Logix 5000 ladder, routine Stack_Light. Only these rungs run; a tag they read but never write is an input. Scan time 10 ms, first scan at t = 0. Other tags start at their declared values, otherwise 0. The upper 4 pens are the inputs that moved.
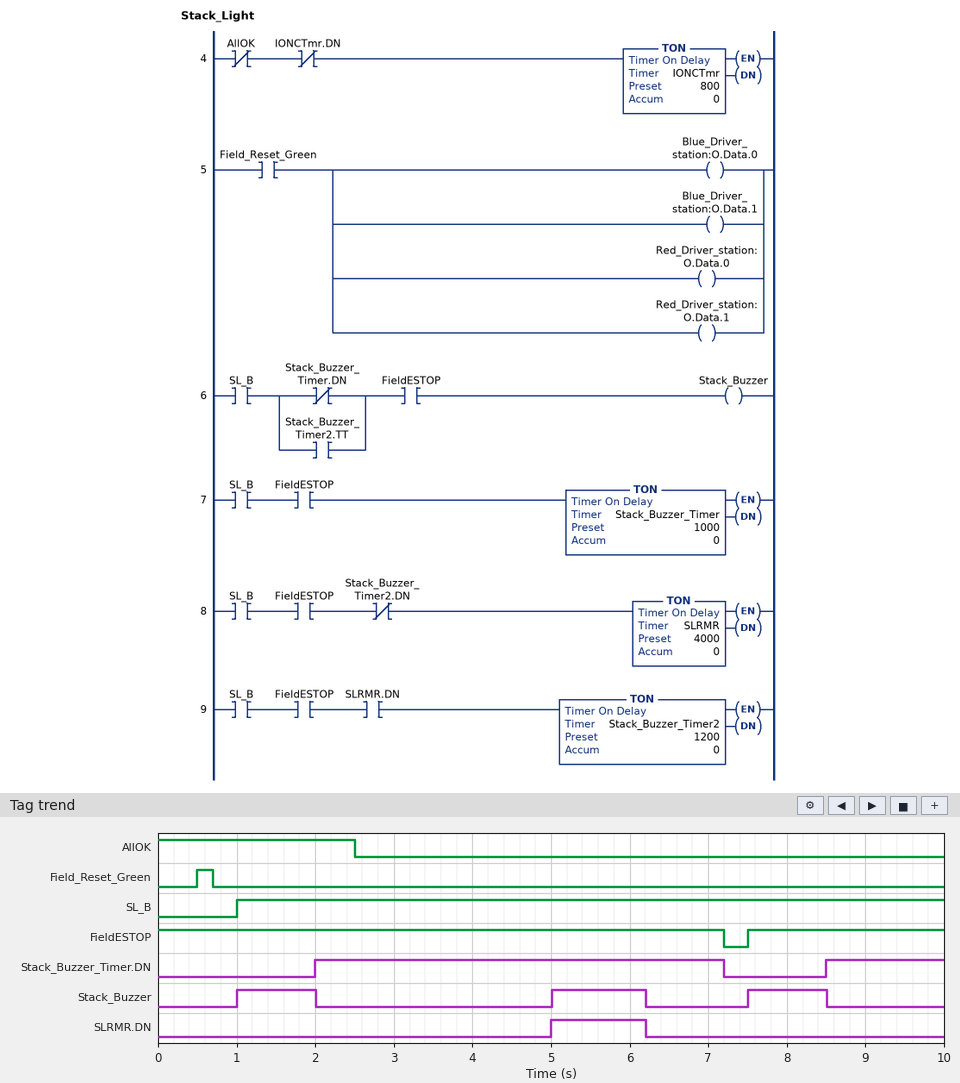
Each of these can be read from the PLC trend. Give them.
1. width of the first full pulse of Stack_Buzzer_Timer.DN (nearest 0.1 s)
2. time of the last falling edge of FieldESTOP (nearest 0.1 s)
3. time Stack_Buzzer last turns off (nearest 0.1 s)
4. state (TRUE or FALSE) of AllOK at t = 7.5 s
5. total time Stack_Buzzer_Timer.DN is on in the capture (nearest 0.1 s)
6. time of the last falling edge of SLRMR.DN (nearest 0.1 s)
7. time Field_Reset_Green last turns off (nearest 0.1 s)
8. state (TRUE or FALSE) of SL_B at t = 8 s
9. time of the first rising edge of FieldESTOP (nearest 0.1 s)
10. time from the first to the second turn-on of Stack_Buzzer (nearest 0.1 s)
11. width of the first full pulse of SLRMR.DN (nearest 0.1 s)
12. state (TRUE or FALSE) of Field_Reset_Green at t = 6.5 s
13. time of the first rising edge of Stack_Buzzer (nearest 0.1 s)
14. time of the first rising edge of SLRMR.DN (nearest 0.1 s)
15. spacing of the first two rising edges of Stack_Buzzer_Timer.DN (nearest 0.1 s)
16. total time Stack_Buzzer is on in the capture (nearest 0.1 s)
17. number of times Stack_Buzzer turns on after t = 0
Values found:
5.2 s
7.2 s
8.5 s
FALSE
6.7 s
6.2 s
0.7 s
TRUE
7.5 s
4.0 s
1.2 s
FALSE
1.0 s
5.0 s
6.5 s
3.2 s
3
